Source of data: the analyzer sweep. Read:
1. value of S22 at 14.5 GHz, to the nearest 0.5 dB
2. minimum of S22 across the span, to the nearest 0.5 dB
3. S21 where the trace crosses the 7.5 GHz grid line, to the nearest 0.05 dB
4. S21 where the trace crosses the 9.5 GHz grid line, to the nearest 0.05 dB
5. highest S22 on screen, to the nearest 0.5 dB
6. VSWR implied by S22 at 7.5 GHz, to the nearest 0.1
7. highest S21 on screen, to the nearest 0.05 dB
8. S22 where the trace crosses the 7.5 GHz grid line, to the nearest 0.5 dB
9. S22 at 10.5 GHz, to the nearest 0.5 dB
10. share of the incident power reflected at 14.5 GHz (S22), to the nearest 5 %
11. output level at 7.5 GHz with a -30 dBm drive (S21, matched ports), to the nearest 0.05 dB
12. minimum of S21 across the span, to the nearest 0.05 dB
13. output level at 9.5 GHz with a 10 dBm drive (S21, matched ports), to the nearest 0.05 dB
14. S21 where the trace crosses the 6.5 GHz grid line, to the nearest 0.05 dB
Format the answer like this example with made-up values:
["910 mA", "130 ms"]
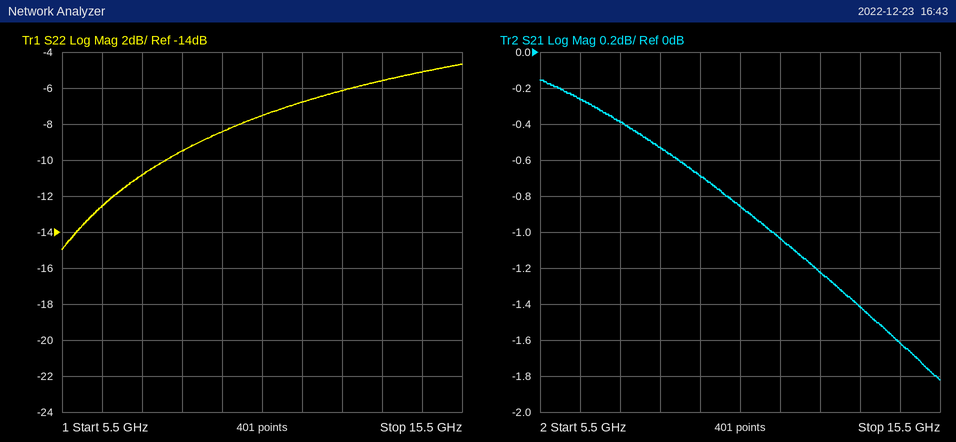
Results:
["-5.0 dB", "-15.0 dB", "-0.40 dB", "-0.70 dB", "-4.5 dB", "1.8", "-0.15 dB", "-11.0 dB", "-7.5 dB", "30 %", "-30.40 dBm", "-1.80 dB", "9.30 dBm", "-0.25 dB"]
